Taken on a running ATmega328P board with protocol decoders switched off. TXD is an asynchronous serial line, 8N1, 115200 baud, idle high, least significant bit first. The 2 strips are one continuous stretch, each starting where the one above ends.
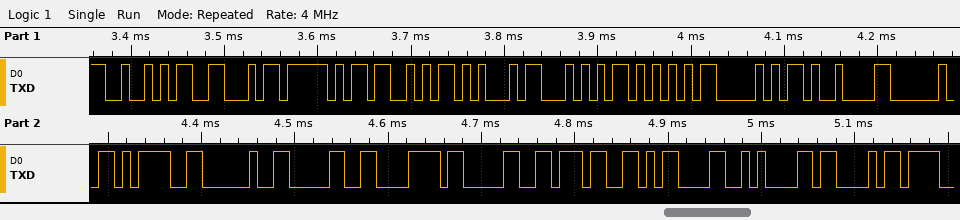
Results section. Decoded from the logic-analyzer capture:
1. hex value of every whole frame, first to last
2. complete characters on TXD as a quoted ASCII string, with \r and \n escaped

52 46 5F 53 45 54 55 50 09 20 3D 20 30 78 30 37 0D 0A 43
"RF_SETUP\t = 0x07\r\nC"
